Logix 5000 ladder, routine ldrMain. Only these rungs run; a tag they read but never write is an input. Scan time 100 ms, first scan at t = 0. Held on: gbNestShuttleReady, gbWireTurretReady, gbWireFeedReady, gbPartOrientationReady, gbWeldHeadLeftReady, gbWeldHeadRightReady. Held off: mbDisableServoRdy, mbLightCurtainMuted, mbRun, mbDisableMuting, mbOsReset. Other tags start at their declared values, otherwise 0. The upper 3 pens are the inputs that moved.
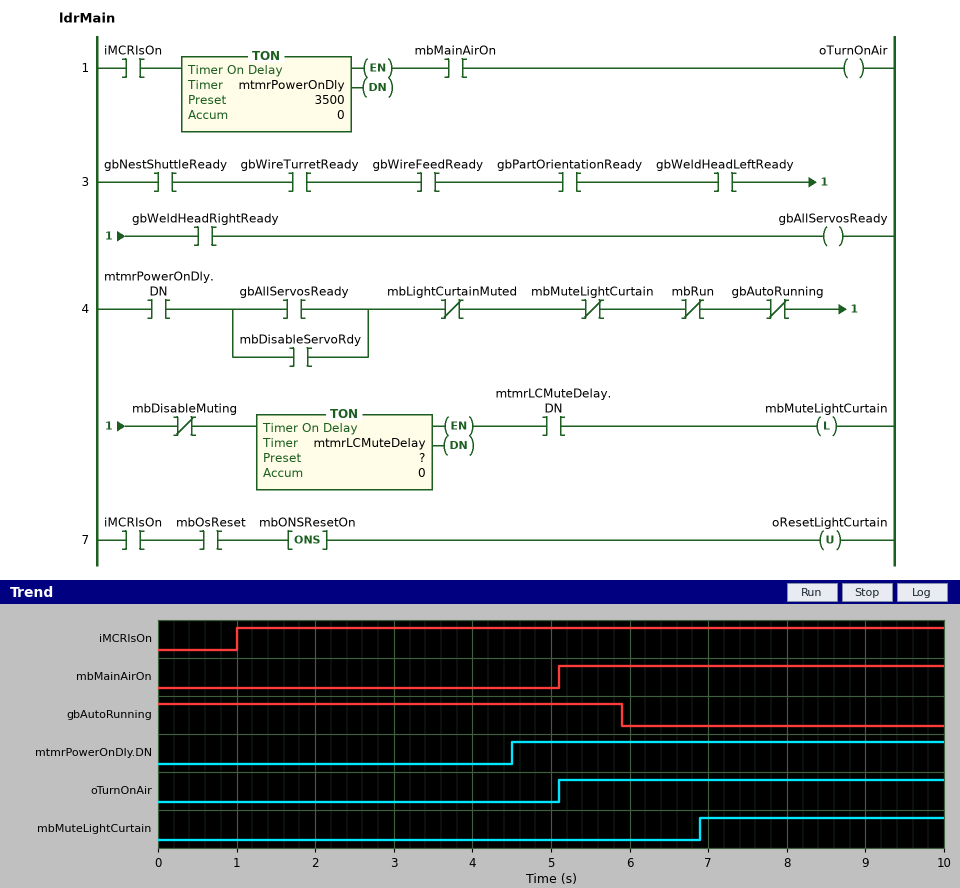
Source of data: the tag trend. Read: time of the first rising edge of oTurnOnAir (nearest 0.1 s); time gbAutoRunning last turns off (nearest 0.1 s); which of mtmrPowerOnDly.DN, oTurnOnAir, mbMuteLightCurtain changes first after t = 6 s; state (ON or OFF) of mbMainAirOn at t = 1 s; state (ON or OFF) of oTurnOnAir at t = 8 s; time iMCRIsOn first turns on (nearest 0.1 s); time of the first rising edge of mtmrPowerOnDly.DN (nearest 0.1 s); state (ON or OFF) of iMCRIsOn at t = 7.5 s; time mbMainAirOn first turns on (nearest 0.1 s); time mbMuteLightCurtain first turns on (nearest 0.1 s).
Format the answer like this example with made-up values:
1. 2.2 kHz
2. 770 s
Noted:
1. 5.1 s
2. 5.9 s
3. mbMuteLightCurtain
4. OFF
5. ON
6. 1.0 s
7. 4.5 s
8. ON
9. 5.1 s
10. 6.9 s
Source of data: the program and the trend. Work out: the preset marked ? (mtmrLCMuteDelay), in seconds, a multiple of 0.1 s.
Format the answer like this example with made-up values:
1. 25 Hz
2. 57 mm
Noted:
1. 1.0 s
